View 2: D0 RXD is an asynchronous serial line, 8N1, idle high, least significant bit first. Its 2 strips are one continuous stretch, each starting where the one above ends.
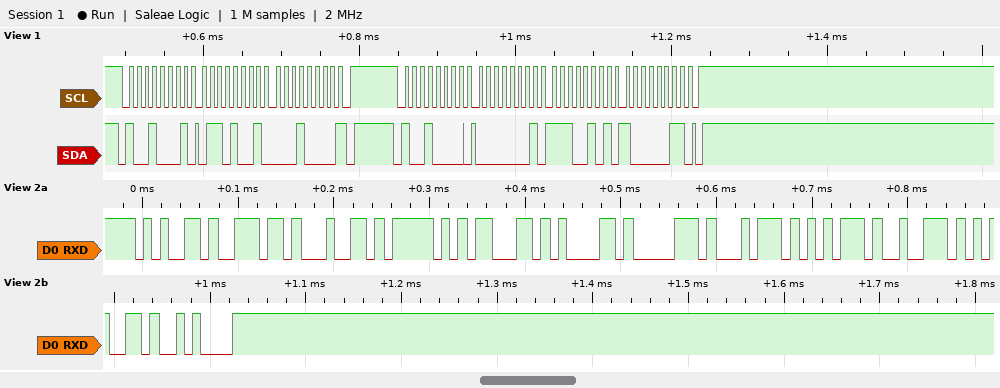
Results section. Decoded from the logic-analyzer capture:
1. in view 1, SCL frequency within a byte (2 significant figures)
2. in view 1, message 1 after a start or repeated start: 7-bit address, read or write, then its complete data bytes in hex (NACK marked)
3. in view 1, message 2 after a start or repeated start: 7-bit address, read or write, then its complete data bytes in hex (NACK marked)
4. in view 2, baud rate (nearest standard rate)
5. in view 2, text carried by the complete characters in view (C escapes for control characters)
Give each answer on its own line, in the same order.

100 kHz
0x48 read: 69 10 NACK
0x48 write: 01 E5 83
115200 baud
"end_capture\n"
